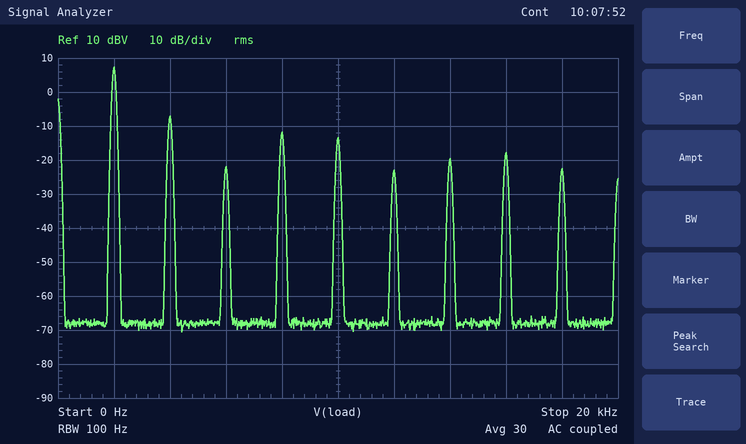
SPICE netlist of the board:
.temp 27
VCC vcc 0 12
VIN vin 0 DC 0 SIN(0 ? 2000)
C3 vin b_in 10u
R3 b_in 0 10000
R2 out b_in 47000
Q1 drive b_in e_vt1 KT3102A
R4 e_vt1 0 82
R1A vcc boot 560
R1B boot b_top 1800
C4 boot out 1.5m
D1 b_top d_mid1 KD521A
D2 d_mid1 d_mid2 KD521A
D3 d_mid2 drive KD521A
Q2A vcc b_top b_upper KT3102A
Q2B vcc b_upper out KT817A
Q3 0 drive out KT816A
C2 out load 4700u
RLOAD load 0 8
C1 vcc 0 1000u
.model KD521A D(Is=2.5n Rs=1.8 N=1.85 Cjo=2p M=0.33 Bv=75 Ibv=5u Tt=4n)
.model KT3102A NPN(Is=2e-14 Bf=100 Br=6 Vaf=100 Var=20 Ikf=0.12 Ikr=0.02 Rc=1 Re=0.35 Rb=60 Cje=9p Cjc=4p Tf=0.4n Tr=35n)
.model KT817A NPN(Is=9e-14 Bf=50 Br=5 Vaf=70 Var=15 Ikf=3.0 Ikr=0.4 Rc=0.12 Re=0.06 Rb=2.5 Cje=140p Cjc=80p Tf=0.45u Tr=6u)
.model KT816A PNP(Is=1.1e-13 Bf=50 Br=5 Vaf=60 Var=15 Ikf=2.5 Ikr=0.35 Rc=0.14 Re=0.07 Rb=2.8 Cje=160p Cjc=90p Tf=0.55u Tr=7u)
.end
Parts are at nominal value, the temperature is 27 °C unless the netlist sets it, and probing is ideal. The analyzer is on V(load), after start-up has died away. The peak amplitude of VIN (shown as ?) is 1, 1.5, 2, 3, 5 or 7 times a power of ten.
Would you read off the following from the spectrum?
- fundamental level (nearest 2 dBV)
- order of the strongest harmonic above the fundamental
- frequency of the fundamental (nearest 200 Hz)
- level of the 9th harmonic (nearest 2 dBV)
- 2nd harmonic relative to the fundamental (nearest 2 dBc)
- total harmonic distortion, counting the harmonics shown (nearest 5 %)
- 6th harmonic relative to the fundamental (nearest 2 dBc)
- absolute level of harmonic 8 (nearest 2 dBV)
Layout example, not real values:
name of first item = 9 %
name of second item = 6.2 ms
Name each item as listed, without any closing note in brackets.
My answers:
fundamental level = 8 dBV
order of the strongest harmonic above the fundamental = 2
frequency of the fundamental = 2.0 kHz
level of the 9th harmonic = -22 dBV
2nd harmonic relative to the fundamental = -14 dBc
total harmonic distortion, counting the harmonics shown = 25 %
6th harmonic relative to the fundamental = -30 dBc
absolute level of harmonic 8 = -18 dBV
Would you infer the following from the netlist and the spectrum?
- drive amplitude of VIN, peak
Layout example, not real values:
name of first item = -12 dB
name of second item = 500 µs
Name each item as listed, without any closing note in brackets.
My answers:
drive amplitude of VIN, peak = 500 mV
